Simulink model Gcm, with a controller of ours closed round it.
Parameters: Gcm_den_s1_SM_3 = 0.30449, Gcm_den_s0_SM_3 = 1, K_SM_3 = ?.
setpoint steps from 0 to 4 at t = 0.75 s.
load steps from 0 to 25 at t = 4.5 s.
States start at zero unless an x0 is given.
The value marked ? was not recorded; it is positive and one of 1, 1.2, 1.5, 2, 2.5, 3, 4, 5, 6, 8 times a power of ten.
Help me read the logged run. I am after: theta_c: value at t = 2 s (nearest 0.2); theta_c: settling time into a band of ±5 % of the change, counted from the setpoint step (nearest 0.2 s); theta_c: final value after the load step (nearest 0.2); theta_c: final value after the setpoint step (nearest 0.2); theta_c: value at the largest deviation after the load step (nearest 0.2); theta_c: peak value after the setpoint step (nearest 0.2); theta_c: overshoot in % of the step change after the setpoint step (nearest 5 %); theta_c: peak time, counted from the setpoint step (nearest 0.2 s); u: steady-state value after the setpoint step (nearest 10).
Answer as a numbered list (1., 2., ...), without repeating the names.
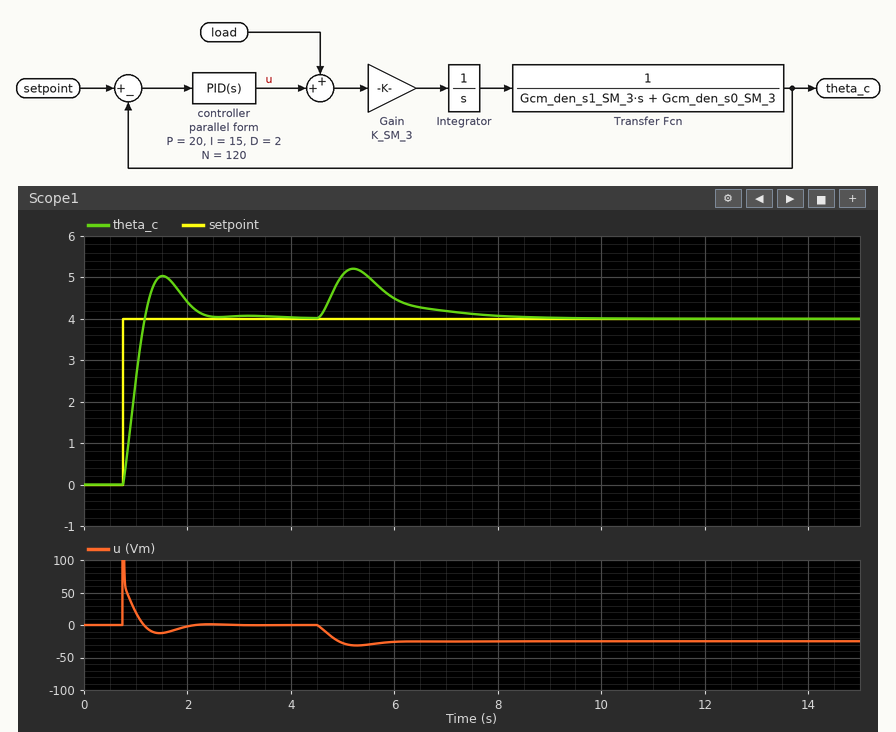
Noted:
1. 4.4
2. 1.4 s
3. 4.0
4. 4.0
5. 5.2
6. 5.0
7. 25 %
8. 0.8 s
9. 0
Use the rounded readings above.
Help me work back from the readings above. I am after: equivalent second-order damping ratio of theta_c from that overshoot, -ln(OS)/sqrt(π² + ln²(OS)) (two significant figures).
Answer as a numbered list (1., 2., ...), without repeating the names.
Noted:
1. 0.40
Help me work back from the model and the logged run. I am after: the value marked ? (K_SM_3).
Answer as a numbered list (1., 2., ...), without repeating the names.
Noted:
1. 0.3
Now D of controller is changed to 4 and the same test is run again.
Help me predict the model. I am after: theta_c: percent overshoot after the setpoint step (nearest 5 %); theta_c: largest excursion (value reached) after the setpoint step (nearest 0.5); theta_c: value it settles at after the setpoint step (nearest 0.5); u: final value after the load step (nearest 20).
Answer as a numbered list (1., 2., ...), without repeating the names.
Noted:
1. 15 %
2. 4.5
3. 4.0
4. -20
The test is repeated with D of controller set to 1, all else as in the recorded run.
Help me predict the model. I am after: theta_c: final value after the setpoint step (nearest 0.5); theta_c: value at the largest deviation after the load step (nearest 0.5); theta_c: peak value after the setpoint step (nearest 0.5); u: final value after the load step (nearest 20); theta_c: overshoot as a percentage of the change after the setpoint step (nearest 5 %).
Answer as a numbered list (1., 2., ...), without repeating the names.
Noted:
1. 4.0
2. 5.5
3. 5.5
4. -20
5. 35 %
